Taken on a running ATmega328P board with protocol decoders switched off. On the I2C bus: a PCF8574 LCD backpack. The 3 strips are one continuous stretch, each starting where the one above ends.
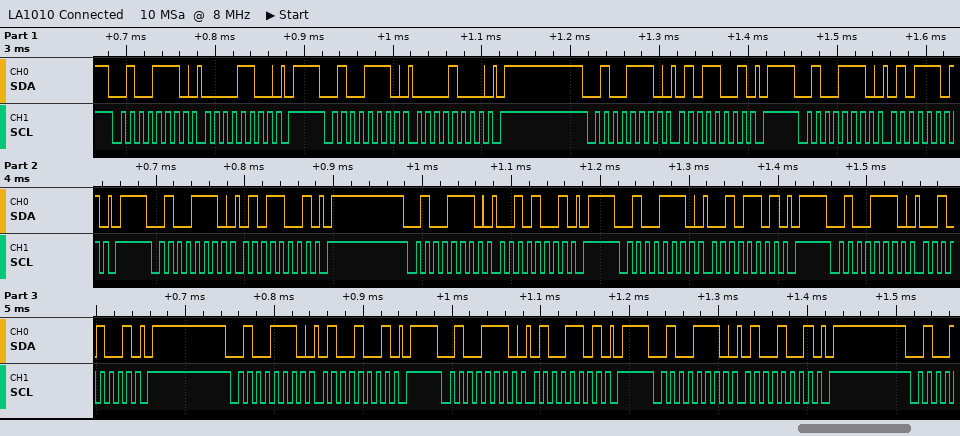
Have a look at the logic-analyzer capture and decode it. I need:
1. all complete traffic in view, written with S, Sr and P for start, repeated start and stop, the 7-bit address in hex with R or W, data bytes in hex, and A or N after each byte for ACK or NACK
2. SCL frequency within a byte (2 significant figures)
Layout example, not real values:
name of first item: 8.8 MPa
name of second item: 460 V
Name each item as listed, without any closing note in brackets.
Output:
all complete traffic in view, written with S, Sr and P for start, repeated start and stop, the 7-bit address in hex with R or W, data bytes in hex, and A or N after each byte for ACK or NACK: S 27W A 0C A P S 27W A 08 A P S 27W A 59 A P S 27W A 5D A P S 27W A 59 A P S 27W A 29 A P S 27W A 2D A P S 27W A 29 A P S 27W A 49 A P S 27W A 4D A P S 27W A 49 A P
SCL frequency within a byte: 100 kHz
